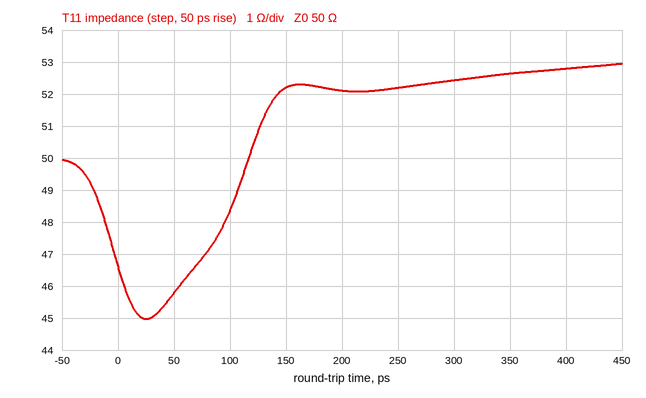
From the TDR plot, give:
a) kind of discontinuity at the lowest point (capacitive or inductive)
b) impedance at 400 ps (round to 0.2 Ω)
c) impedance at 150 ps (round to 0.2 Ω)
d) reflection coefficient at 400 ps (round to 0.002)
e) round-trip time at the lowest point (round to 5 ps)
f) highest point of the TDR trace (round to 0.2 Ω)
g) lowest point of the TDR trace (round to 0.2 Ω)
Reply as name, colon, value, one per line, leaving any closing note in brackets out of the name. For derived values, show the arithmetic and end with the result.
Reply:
kind of discontinuity at the lowest point: capacitive
impedance at 400 ps: 52.8 Ω
impedance at 150 ps: 52.2 Ω
reflection coefficient at 400 ps: (52.8 − 50)/(52.8 + 50) ≈ +0.0272, so +0.028 to the nearest 0.002
round-trip time at the lowest point: 25 ps
highest point of the TDR trace: 53.0 Ω
lowest point of the TDR trace: 45.0 Ω
